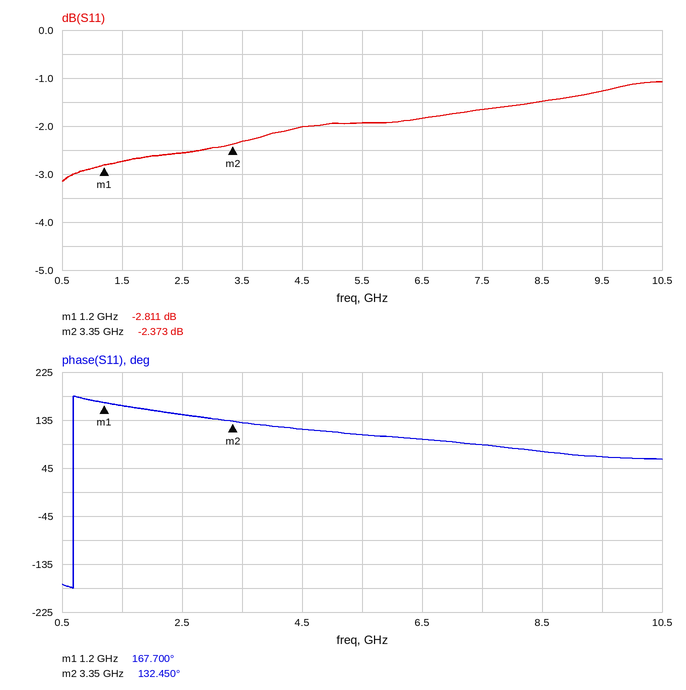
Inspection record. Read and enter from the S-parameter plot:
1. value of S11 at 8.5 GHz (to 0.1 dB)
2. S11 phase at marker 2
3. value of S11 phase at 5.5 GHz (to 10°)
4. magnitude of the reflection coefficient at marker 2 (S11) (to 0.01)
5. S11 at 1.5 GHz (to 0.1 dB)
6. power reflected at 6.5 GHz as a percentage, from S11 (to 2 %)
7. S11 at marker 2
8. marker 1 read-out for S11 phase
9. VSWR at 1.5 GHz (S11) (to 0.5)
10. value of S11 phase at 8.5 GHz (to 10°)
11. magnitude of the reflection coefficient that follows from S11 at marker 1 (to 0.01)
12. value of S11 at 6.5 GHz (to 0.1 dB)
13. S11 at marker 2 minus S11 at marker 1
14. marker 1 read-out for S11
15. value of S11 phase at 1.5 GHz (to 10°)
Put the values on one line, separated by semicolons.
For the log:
-1.5 dB; 132.450°; 110°; 0.76; -2.7 dB; 66 %; -2.373 dB; 167.700°; 6.5; 80°; 0.72; -1.8 dB; 0.438 dB; -2.811 dB; 160°
